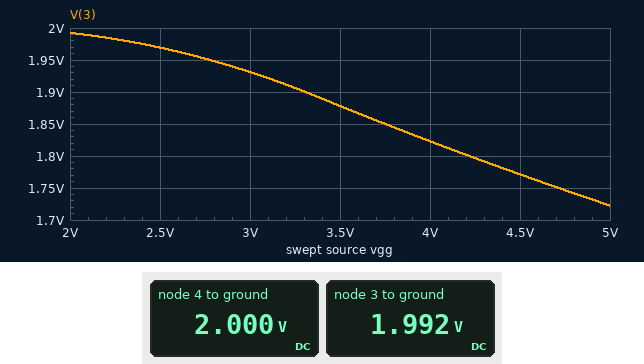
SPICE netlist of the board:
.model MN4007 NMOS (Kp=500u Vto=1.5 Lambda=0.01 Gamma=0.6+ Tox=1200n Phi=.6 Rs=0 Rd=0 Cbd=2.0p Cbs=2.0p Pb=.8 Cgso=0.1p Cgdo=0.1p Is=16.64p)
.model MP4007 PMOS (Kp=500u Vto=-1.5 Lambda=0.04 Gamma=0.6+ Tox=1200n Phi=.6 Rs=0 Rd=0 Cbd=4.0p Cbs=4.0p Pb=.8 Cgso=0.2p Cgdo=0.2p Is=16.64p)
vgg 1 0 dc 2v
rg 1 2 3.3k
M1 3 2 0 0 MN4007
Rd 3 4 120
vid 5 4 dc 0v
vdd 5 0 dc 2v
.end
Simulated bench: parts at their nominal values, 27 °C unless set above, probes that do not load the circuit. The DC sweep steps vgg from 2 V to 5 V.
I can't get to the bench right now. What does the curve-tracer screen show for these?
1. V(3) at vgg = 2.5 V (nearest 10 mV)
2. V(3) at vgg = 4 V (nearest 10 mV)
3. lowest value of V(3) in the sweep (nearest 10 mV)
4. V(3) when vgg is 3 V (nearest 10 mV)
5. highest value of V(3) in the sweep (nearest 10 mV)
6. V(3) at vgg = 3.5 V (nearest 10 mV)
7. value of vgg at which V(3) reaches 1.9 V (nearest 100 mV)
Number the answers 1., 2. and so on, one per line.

1. 1.97 V
2. 1.82 V
3. 1.72 V
4. 1.93 V
5. 1.99 V
6. 1.88 V
7. 3.3 V
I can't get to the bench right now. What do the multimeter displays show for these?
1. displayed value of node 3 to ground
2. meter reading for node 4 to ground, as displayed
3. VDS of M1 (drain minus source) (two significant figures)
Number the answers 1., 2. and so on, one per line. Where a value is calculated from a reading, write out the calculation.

1. 1.992 V
2. 2.000 V
3. 1.992 V = 2.0 V
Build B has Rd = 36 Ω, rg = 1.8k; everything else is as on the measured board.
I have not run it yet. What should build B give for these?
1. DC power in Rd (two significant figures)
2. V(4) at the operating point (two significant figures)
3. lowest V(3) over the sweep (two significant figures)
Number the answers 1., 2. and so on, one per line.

1. 150 nW
2. 2.0 V
3. 1.9 V
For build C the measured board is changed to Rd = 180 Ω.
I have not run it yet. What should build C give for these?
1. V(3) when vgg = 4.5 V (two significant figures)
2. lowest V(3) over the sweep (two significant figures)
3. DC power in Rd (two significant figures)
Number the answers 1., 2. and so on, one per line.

1. 1.7 V
2. 1.6 V
3. 730 nW
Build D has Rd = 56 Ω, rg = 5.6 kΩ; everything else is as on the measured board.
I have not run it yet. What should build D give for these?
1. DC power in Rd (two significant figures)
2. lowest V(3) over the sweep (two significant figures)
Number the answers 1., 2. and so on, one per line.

1. 230 nW
2. 1.9 V
